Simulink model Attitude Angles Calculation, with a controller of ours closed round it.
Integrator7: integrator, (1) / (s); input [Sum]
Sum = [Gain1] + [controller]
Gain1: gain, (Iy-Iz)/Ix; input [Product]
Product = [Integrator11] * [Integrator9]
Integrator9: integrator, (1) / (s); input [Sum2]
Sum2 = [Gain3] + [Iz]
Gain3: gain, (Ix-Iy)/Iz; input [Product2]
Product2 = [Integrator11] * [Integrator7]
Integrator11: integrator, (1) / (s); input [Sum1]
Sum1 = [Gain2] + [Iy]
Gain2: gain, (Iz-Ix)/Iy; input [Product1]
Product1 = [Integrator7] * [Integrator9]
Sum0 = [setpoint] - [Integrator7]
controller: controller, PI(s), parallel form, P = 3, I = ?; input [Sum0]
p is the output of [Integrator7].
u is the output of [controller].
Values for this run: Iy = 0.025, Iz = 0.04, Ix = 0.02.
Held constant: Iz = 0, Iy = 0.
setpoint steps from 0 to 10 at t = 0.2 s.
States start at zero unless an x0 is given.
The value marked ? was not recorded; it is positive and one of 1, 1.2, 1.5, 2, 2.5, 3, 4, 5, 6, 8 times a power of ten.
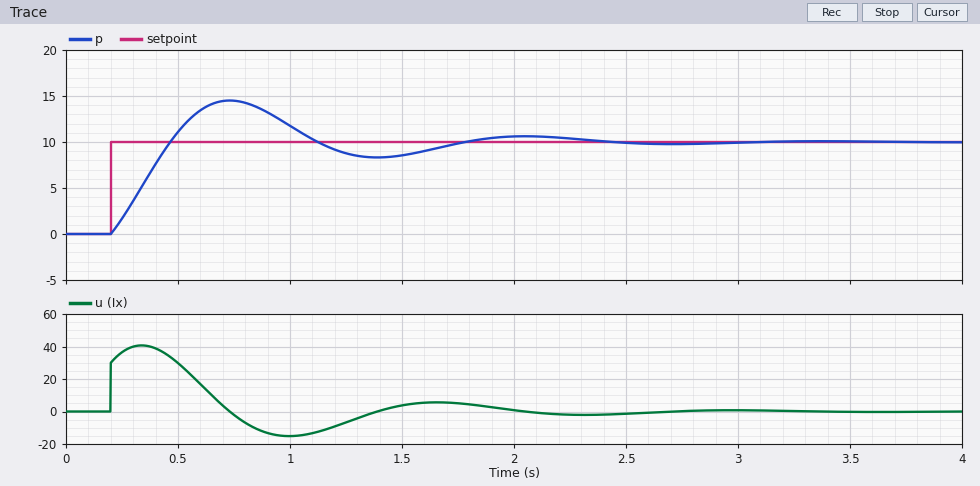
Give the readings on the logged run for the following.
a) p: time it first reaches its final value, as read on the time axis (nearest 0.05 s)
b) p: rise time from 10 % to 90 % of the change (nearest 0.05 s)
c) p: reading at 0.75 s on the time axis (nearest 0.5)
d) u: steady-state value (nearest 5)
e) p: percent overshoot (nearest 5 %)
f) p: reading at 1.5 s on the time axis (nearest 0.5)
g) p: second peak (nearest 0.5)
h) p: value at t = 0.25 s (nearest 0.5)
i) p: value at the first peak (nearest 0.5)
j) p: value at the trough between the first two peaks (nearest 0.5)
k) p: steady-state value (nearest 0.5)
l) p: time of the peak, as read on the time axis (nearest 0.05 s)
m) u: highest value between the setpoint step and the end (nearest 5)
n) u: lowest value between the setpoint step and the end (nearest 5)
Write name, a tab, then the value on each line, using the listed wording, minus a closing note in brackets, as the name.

p: time it first reaches its final value, as read on the time axis	0.45 s
p: rise time from 10 % to 90 % of the change	0.20 s
p: reading at 0.75 s on the time axis	14.5
u: steady-state value	0
p: percent overshoot	45 %
p: reading at 1.5 s on the time axis	8.5
p: second peak	10.5
p: value at t = 0.25 s	1.5
p: value at the first peak	14.5
p: value at the trough between the first two peaks	8.5
p: steady-state value	10.0
p: time of the peak, as read on the time axis	0.75 s
u: highest value between the setpoint step and the end	40
u: lowest value between the setpoint step and the end	-15
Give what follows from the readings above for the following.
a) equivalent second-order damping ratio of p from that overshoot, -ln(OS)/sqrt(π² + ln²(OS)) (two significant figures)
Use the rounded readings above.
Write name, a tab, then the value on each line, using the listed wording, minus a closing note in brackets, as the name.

equivalent second-order damping ratio of p from that overshoot, -ln(OS)/sqrt(π² + ln²(OS))	0.25
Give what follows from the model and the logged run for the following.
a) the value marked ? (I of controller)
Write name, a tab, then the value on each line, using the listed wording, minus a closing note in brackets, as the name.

the value marked ?	25
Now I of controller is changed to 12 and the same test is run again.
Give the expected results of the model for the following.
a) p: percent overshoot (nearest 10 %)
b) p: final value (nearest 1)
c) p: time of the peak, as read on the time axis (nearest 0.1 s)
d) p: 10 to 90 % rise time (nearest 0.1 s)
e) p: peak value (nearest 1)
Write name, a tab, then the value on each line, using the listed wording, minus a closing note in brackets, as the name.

p: percent overshoot	30 %
p: final value	10
p: time of the peak, as read on the time axis	0.9 s
p: 10 to 90 % rise time	0.3 s
p: peak value	13
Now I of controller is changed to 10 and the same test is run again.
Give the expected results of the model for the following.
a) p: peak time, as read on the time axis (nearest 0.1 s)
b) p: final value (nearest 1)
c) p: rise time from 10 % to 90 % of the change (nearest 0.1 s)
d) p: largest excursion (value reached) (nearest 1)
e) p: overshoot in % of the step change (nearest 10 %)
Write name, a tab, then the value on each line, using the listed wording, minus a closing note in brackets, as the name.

p: peak time, as read on the time axis	1.0 s
p: final value	10
p: rise time from 10 % to 90 % of the change	0.3 s
p: largest excursion (value reached)	13
p: overshoot in % of the step change	30 %
